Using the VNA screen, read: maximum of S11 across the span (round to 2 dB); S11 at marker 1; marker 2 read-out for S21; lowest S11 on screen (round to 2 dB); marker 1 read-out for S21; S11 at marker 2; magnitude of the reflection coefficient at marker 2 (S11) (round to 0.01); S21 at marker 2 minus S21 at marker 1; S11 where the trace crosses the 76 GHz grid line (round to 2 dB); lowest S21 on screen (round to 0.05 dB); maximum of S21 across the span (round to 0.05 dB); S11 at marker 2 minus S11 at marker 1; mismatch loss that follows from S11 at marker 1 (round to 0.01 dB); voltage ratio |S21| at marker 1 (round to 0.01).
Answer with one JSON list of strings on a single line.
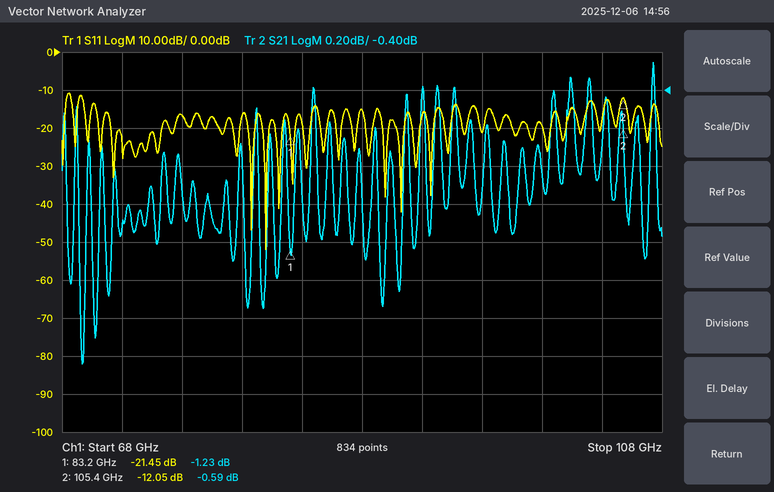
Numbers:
["-10 dB", "-21.45 dB", "-0.59 dB", "-52 dB", "-1.23 dB", "-12.05 dB", "0.25", "0.64 dB", "-16 dB", "-1.85 dB", "-0.25 dB", "9.40 dB", "0.03 dB", "0.87"]
